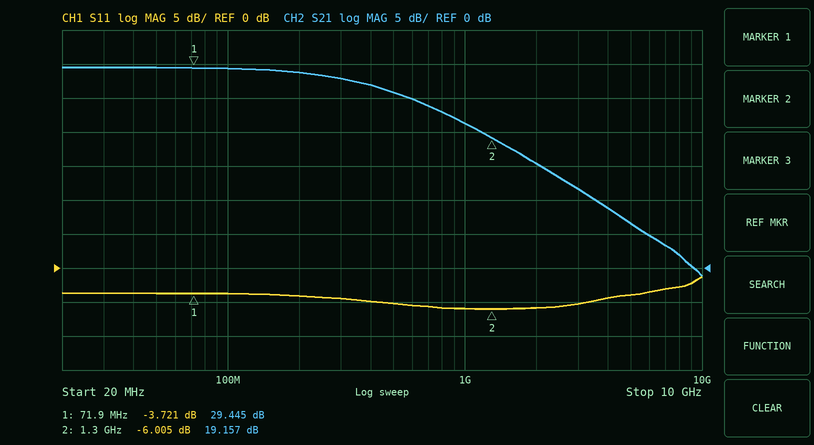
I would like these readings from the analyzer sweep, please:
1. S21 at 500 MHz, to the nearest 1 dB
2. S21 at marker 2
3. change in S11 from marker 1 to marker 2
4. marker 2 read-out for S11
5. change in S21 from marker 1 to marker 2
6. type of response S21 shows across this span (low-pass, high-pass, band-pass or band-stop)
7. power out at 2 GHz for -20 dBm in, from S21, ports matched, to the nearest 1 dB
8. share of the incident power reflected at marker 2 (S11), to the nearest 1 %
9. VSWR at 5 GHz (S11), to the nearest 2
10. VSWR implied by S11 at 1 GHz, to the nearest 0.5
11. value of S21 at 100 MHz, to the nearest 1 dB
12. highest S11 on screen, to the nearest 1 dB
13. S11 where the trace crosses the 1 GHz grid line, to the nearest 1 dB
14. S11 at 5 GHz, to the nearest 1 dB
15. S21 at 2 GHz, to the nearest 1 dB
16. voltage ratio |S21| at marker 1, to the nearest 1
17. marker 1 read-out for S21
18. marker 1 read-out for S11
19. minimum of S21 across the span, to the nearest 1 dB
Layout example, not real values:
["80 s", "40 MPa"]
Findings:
["26 dB", "19.157 dB", "-2.284 dB", "-6.005 dB", "-10.288 dB", "low-pass", "-5 dBm", "25 %", "4", "3.0", "29 dB", "-1 dB", "-6 dB", "-4 dB", "15 dB", "30", "29.445 dB", "-3.721 dB", "-1 dB"]
